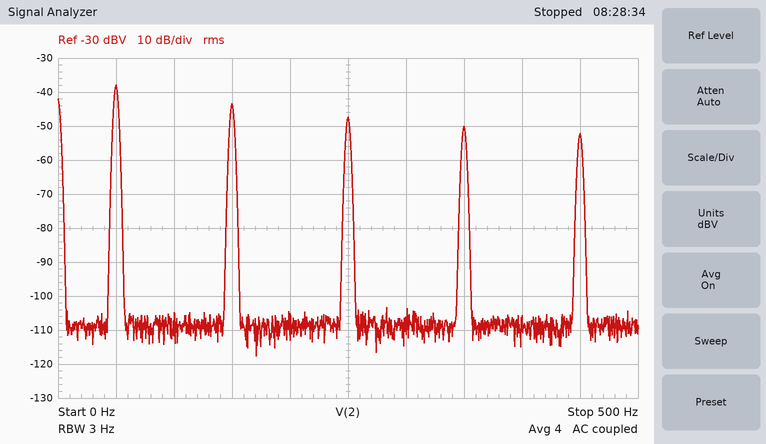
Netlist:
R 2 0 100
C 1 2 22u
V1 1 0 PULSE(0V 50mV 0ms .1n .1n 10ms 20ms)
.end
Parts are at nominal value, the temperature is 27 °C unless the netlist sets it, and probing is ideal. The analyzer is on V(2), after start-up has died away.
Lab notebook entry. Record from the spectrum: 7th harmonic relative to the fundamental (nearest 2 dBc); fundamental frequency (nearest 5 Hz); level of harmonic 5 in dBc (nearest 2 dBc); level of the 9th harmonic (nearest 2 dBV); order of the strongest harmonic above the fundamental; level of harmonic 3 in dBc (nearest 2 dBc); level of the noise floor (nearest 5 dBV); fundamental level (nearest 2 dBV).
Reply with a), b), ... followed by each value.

a) -12 dBc
b) 50 Hz
c) -10 dBc
d) -52 dBV
e) 3
f) -6 dBc
g) -110 dBV
h) -38 dBV
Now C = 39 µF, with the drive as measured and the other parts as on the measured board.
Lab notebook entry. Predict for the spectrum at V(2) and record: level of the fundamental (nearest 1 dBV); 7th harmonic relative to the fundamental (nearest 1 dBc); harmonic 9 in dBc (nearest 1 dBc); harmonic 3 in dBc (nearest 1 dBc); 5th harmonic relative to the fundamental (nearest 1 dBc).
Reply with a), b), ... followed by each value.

a) -35 dBV
b) -15 dBc
c) -17 dBc
d) -8 dBc
e) -12 dBc
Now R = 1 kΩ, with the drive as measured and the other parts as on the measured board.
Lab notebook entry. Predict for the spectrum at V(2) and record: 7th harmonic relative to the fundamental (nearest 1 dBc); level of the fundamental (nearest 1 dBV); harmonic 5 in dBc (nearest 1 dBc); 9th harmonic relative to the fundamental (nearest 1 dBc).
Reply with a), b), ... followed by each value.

a) -17 dBc
b) -33 dBV
c) -14 dBc
d) -19 dBc
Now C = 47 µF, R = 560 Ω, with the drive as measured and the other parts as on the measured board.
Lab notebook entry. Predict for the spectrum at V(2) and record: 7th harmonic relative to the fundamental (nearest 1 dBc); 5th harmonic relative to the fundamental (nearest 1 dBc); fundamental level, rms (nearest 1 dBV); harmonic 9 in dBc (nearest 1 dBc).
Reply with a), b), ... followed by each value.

a) -17 dBc
b) -14 dBc
c) -33 dBV
d) -19 dBc
